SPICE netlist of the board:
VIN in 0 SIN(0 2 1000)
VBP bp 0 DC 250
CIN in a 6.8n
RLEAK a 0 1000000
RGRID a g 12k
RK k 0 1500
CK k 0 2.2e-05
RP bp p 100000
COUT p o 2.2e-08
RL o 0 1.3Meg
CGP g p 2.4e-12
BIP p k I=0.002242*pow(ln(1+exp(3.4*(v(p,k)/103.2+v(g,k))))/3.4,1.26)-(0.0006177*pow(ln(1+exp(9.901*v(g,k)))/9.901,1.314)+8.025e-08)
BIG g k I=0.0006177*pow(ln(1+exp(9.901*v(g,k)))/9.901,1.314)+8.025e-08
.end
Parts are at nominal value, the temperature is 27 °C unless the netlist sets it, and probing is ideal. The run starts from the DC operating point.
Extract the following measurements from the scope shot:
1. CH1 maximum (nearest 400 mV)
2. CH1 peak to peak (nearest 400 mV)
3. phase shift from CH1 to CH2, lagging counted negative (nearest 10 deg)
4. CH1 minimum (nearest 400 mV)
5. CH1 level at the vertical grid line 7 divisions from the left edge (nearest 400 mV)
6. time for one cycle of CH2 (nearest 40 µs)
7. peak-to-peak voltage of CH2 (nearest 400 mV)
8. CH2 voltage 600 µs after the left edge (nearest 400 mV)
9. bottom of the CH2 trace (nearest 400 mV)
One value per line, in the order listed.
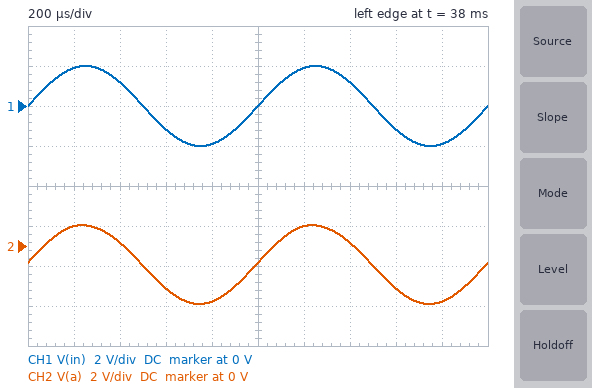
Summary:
2.0 V
4.0 V
0 deg
-2.0 V
1.2 V
1.00 ms
4.0 V
-2.0 V
-2.8 V
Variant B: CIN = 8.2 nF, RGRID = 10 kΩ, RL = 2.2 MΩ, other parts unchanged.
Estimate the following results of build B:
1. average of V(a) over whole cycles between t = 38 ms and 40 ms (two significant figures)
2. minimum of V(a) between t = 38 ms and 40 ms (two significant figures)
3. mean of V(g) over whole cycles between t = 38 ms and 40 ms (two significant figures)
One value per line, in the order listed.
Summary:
-940 mV
-2.9 V
-950 mV
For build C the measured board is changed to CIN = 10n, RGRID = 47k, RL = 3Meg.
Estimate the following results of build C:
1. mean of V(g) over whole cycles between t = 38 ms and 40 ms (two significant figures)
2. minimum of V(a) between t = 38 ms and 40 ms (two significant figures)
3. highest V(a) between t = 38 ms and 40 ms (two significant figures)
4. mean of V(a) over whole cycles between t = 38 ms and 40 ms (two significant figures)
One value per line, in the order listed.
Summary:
-830 mV
-2.8 V
1.2 V
-790 mV
